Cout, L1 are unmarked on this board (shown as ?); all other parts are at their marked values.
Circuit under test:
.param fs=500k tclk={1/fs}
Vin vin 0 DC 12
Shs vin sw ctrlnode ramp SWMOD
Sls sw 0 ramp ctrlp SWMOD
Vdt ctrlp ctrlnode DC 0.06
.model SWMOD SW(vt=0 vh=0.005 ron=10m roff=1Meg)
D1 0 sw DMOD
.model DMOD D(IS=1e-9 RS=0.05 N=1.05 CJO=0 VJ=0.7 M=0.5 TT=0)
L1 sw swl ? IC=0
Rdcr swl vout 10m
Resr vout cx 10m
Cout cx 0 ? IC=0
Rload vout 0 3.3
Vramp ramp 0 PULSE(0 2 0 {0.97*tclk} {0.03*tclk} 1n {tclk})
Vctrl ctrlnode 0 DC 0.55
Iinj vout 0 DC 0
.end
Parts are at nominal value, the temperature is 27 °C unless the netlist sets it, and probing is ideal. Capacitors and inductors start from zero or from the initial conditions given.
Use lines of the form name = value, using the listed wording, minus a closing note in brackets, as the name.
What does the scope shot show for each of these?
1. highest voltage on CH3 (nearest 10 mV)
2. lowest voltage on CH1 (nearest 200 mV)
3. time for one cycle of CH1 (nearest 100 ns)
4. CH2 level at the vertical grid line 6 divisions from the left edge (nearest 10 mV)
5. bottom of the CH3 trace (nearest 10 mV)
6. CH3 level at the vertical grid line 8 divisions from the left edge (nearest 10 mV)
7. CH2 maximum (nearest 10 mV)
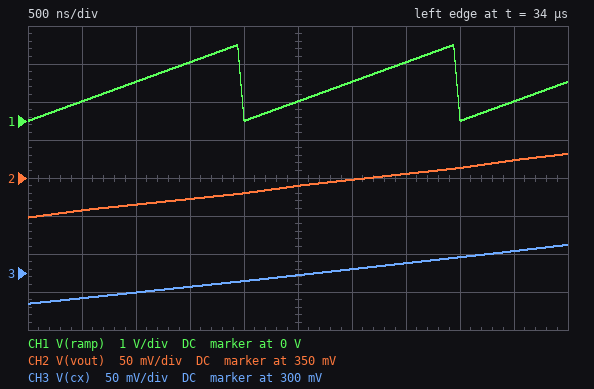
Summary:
highest voltage on CH3 = 340 mV
lowest voltage on CH1 = 0 V
time for one cycle of CH1 = 2.0 µs
CH2 level at the vertical grid line 6 divisions from the left edge = 350 mV
bottom of the CH3 trace = 260 mV
CH3 level at the vertical grid line 8 divisions from the left edge = 320 mV
CH2 maximum = 380 mV
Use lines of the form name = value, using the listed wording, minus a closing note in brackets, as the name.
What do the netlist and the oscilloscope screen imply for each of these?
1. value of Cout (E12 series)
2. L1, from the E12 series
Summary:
value of Cout = 270 µF
L1, from the E12 series = 27 µH
